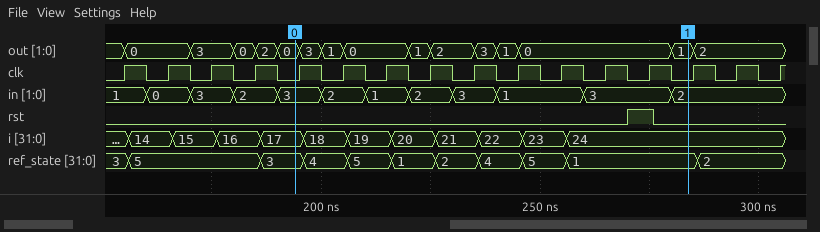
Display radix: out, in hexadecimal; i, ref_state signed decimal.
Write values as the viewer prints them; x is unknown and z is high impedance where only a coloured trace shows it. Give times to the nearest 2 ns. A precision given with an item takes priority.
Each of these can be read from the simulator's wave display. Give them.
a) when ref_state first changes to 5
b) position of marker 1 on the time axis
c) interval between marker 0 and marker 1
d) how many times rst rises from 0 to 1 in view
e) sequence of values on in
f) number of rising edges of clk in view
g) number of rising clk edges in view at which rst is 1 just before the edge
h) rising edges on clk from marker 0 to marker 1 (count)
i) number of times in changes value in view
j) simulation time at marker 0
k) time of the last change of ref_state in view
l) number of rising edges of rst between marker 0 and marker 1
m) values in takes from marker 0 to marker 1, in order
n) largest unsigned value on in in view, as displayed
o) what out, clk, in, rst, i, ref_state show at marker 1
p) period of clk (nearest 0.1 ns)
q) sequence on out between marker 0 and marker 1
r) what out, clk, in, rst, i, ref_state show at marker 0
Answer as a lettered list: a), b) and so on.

a) 156 ns
b) 284 ns
c) 90 ns
d) 1
e) 1, 0, 3, 2, 3, 2, 1, 2, 3, 1, 3, 2
f) 16
g) 1
h) 9
i) 11
j) 194 ns
k) 286 ns
l) 1
m) 3, 2, 1, 2, 3, 1, 3, 2
n) 3
o) out=1, clk=0, in=2, rst=0, i=24, ref_state=1
p) 10 ns
q) 0, 3, 1, 0, 1, 2, 3, 1, 0, 1
r) out=0, clk=0, in=3, rst=0, i=17, ref_state=3
